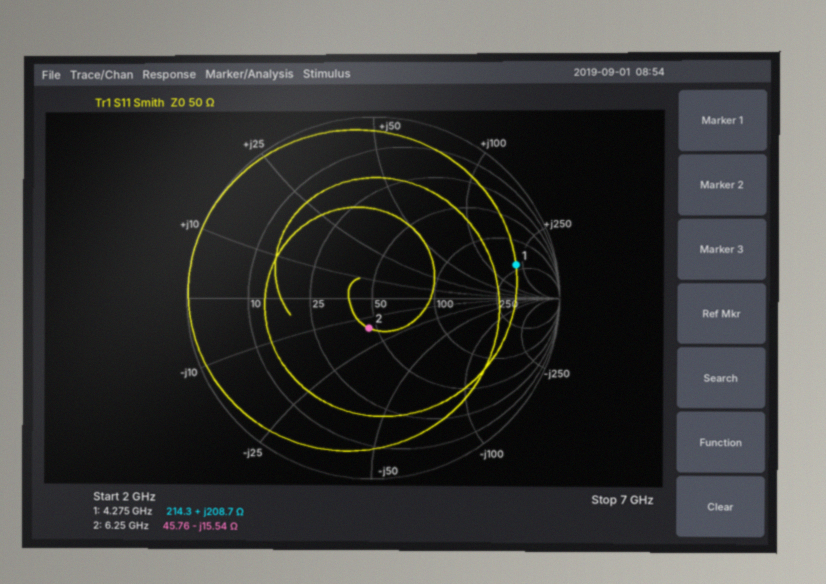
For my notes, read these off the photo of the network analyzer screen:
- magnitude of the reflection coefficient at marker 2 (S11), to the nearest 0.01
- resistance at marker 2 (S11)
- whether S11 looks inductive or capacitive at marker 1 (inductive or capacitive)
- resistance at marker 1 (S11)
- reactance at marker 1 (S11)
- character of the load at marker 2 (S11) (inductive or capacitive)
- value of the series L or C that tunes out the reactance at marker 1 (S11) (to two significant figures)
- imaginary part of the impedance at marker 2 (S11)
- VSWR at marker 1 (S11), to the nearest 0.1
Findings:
0.17
45.76 Ω
inductive
214.3 Ω
+208.7 Ω
capacitive
180 fF
-15.54 Ω
8.5
